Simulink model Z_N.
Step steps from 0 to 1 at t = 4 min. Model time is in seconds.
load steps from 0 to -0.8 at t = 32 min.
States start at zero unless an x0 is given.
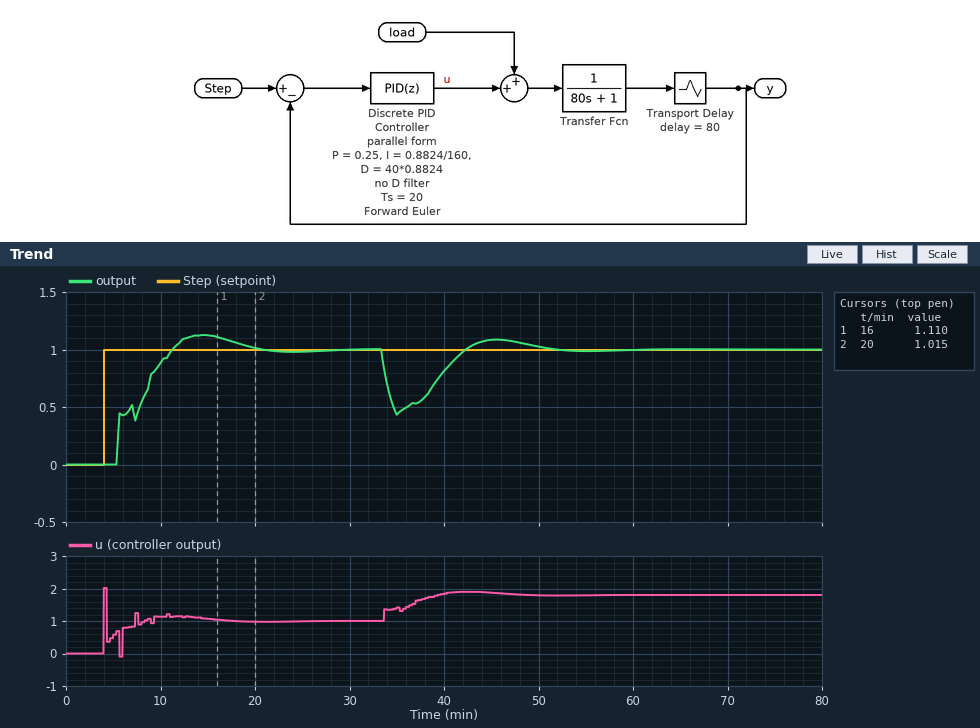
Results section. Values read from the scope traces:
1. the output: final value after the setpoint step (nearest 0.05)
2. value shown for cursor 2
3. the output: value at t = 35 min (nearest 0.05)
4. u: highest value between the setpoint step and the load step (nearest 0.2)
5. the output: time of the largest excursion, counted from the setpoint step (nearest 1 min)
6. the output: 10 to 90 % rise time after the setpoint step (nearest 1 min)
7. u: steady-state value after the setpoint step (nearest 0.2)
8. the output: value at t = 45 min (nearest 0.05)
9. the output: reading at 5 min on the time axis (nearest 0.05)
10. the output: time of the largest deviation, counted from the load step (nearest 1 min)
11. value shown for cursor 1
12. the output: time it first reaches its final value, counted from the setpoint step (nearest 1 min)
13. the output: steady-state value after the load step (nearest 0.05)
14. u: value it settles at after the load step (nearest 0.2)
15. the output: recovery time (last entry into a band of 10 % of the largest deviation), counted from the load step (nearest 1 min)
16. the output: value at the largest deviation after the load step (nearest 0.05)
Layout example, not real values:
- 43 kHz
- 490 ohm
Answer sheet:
- 1.00
- 1.015
- 0.45
- 2.0
- 11 min
- 5 min
- 1.0
- 1.10
- 0.00
- 3 min
- 1.110
- 7 min
- 1.00
- 1.8
- 16 min
- 0.45
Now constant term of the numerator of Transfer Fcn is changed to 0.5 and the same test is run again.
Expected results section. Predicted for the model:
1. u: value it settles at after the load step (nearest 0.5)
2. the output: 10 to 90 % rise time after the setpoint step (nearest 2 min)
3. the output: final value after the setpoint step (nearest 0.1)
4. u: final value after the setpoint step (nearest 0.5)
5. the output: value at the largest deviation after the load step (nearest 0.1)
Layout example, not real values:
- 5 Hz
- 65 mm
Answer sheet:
- 3.0
- 10 min
- 1.0
- 2.0
- 0.7
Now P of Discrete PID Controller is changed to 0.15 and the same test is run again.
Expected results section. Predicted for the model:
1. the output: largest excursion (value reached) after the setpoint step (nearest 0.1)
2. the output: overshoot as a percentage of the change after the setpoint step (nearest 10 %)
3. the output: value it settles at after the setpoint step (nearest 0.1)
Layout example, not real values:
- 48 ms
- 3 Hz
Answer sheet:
- 1.2
- 20 %
- 1.0
